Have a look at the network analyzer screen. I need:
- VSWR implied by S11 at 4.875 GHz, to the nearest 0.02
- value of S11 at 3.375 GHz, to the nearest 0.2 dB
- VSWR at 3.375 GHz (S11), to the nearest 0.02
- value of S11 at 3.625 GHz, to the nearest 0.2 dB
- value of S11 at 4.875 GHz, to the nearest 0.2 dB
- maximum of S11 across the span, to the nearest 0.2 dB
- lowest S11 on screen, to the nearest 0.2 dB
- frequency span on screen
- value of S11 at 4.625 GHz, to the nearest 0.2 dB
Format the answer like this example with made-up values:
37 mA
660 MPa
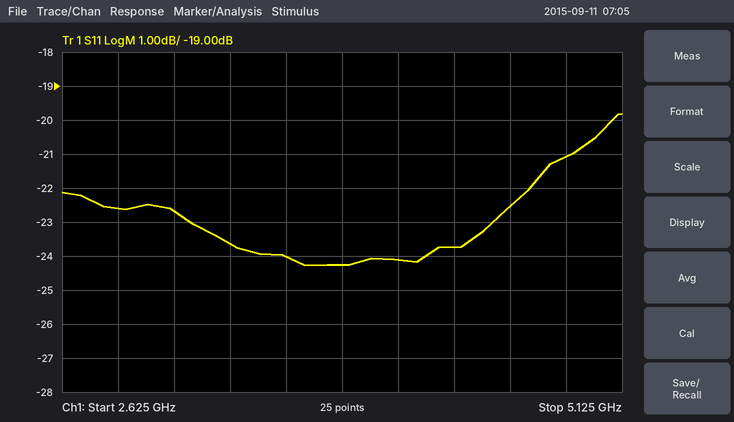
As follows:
1.20
-23.6 dB
1.14
-24.0 dB
-21.0 dB
-19.8 dB
-24.2 dB
2.5 GHz
-22.6 dB
